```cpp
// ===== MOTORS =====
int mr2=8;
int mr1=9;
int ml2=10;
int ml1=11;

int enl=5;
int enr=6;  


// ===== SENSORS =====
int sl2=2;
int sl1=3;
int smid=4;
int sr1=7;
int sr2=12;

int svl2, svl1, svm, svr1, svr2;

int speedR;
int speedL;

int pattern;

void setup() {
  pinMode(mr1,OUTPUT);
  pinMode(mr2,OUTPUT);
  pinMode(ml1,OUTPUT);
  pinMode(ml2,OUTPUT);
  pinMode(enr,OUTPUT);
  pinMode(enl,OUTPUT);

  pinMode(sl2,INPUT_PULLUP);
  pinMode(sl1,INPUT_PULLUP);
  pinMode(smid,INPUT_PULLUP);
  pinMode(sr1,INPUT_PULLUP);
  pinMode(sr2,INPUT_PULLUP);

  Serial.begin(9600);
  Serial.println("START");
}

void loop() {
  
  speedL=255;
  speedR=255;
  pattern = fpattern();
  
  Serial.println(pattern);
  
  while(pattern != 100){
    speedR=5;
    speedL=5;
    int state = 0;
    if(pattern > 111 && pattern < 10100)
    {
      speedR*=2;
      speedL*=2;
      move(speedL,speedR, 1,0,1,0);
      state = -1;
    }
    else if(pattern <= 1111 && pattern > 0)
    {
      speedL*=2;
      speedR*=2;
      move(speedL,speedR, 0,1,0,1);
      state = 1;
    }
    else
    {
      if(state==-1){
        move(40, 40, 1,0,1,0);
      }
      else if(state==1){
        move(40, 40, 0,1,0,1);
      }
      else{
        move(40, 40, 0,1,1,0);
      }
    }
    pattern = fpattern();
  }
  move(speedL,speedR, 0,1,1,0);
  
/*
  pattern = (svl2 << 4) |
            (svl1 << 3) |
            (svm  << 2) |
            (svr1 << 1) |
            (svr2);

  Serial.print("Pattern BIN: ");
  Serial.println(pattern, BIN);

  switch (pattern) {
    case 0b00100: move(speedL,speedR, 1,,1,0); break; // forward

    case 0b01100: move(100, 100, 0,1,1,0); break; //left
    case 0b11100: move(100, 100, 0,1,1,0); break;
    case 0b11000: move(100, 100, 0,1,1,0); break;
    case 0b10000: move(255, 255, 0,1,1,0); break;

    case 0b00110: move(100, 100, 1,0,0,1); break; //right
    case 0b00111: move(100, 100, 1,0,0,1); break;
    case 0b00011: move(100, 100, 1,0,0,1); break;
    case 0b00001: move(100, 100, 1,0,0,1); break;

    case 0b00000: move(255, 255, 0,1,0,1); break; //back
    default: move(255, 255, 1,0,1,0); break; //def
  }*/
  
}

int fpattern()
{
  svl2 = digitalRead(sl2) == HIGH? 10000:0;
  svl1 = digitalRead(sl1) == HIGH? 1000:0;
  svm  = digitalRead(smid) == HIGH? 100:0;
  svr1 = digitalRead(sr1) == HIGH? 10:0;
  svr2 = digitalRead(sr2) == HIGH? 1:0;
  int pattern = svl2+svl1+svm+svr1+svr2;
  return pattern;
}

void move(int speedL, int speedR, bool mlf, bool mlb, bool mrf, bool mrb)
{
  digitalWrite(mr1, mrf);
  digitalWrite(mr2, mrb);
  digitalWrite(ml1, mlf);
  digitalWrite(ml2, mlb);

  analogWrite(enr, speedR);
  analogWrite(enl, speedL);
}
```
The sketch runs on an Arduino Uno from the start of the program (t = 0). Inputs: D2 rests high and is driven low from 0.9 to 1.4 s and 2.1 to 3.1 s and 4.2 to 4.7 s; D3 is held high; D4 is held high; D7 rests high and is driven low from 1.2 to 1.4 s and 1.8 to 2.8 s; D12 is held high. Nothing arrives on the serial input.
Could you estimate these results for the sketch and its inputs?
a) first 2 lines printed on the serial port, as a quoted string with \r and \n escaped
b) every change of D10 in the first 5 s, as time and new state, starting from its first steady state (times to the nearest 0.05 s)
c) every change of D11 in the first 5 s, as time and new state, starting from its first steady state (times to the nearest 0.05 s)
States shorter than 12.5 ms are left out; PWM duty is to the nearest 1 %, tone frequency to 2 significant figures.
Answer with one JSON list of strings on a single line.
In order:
["\"START\\r\\n11111\\r\\n\"", "0 s high; 0.9 s low; 1.4 s high; 2.1 s low; 3.1 s high; 4.2 s low; 4.7 s high", "0 s low; 0.9 s high; 1.4 s low; 2.1 s high; 3.1 s low; 4.2 s high; 4.7 s low"]
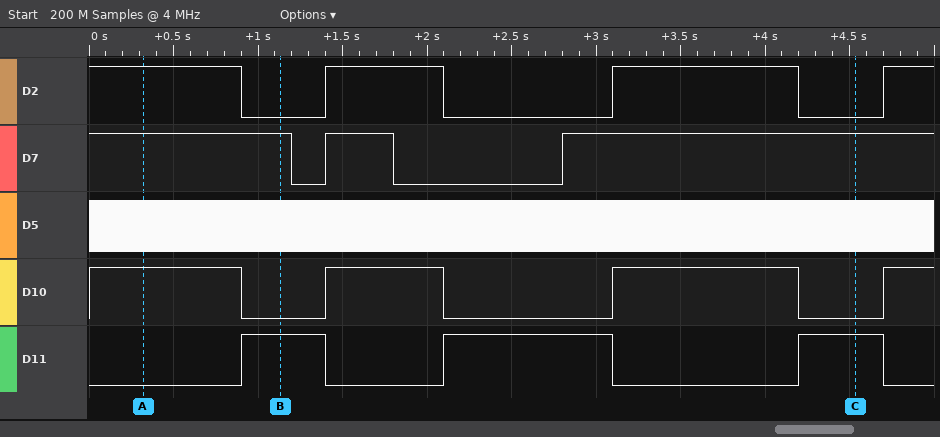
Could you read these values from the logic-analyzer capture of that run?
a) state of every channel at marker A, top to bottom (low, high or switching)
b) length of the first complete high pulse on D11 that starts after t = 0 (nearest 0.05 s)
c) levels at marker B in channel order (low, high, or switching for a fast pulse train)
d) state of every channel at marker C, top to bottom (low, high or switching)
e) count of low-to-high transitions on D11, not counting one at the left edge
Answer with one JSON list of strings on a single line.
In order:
["D2 high, D7 high, D5 switching, D10 high, D11 low", "0.50 s", "D2 low, D7 high, D5 switching, D10 low, D11 high", "D2 low, D7 high, D5 switching, D10 low, D11 high", "3"]
